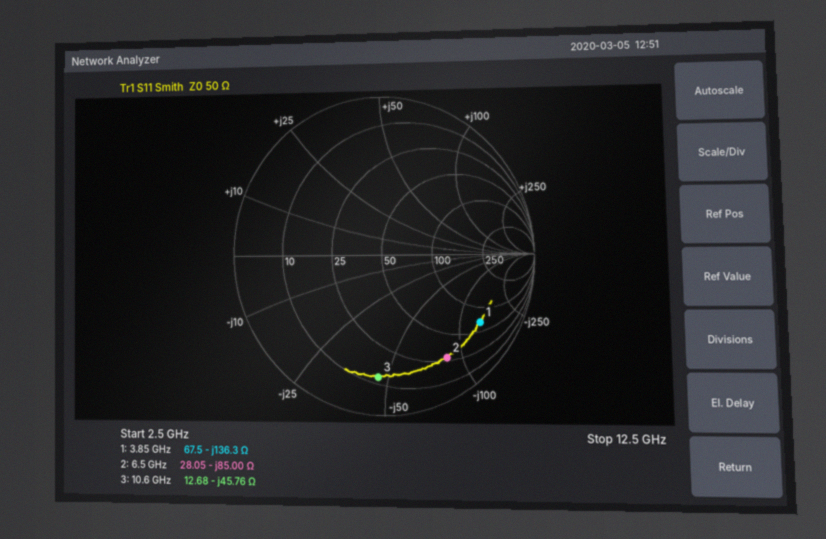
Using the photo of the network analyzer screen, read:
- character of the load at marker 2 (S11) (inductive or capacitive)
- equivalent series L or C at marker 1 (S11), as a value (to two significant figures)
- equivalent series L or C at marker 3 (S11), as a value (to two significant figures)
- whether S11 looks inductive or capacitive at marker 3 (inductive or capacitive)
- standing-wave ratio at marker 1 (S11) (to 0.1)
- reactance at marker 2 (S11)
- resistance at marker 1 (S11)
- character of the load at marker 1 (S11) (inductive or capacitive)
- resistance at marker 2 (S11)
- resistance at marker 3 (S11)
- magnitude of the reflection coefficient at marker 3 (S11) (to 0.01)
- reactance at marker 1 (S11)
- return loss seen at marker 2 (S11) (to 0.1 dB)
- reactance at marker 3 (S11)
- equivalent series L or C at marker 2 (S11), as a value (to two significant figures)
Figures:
capacitive
300 fF
330 fF
capacitive
7.5
-85.00 Ω
67.5 Ω
capacitive
28.05 Ω
12.68 Ω
0.76
-136.3 Ω
2.4 dB
-45.76 Ω
290 fF
